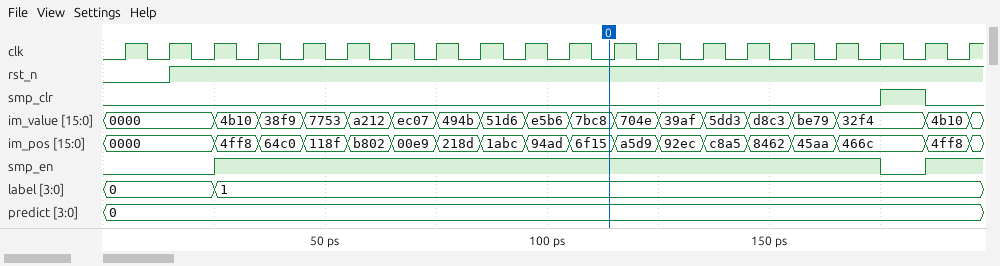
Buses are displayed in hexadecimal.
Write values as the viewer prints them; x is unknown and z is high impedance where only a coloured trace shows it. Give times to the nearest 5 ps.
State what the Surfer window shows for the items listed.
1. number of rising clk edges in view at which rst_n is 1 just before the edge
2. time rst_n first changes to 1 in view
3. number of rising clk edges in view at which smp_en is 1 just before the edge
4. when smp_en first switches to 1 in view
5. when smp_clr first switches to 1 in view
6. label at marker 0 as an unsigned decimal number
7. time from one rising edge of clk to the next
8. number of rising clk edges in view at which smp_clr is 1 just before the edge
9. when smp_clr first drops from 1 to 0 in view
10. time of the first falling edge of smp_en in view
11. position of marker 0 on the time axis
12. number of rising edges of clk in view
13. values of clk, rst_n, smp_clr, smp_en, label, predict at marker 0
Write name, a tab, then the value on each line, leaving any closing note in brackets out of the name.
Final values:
number of rising clk edges in view at which rst_n is 1 just before the edge	18
time rst_n first changes to 1 in view	15 ps
number of rising clk edges in view at which smp_en is 1 just before the edge	16
when smp_en first switches to 1 in view	25 ps
when smp_clr first switches to 1 in view	175 ps
label at marker 0 as an unsigned decimal number	1
time from one rising edge of clk to the next	10 ps
number of rising clk edges in view at which smp_clr is 1 just before the edge	1
when smp_clr first drops from 1 to 0 in view	185 ps
time of the first falling edge of smp_en in view	175 ps
position of marker 0 on the time axis	115 ps
number of rising edges of clk in view	20
values of clk, rst_n, smp_clr, smp_en, label, predict at marker 0	clk=0, rst_n=1, smp_clr=0, smp_en=1, label=1, predict=0
